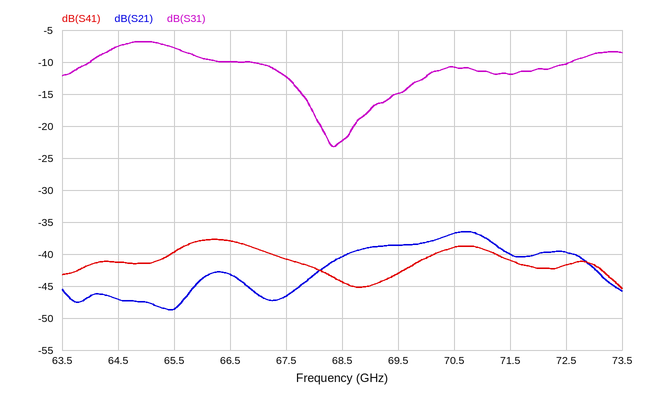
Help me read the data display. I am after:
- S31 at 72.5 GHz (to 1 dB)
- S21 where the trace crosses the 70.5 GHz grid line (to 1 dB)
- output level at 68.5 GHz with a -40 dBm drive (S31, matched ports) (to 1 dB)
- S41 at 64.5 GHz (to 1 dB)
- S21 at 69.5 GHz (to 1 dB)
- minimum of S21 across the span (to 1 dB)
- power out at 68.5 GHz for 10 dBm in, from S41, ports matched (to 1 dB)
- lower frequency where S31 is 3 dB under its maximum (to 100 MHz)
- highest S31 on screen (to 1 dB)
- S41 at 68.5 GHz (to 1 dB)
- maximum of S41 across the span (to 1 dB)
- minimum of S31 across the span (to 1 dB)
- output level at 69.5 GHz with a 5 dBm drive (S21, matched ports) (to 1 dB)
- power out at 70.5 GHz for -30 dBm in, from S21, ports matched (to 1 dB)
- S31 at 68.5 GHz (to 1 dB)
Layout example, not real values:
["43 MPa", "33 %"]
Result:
["-10 dB", "-37 dB", "-62 dBm", "-41 dB", "-39 dB", "-49 dB", "-34 dBm", "64.0 GHz", "-7 dB", "-44 dB", "-38 dB", "-23 dB", "-34 dBm", "-67 dBm", "-22 dB"]
